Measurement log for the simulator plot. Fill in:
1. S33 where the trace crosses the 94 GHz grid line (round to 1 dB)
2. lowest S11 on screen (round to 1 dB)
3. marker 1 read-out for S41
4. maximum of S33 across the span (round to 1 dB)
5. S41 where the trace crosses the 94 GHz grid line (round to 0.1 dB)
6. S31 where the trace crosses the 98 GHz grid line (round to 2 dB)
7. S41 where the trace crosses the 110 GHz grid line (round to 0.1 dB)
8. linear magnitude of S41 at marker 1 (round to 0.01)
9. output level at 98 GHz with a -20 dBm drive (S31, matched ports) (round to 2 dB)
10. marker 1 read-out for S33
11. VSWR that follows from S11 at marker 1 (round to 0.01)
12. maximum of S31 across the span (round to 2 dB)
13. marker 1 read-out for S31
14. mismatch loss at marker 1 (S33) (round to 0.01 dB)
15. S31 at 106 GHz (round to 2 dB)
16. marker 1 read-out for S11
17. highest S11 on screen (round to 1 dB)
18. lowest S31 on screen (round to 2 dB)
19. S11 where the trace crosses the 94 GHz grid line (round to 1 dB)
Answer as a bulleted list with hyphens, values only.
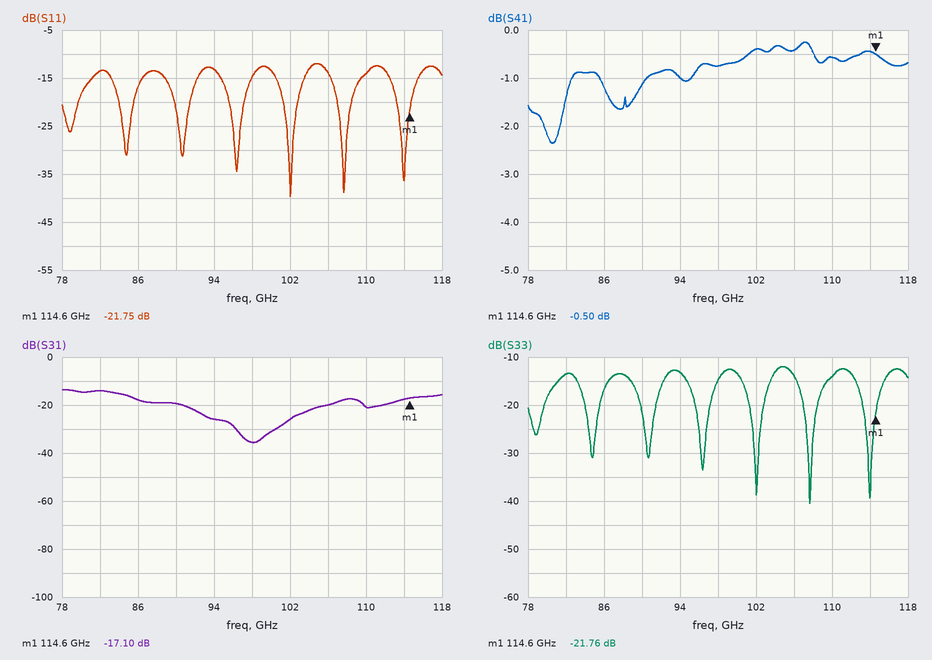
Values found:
- -13 dB
- -40 dB
- -0.50 dB
- -12 dB
- -1.0 dB
- -36 dB
- -0.6 dB
- 0.94
- -56 dBm
- -21.76 dB
- 1.18
- -14 dB
- -17.10 dB
- 0.03 dB
- -20 dB
- -21.75 dB
- -12 dB
- -36 dB
- -13 dB
